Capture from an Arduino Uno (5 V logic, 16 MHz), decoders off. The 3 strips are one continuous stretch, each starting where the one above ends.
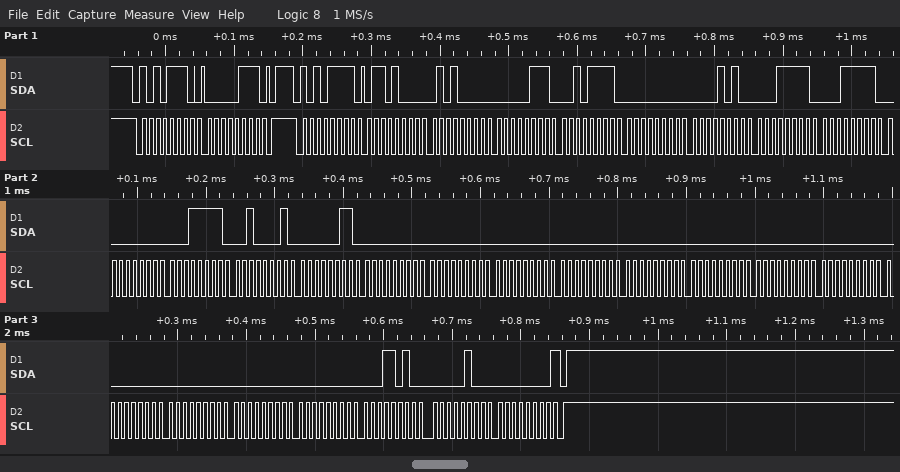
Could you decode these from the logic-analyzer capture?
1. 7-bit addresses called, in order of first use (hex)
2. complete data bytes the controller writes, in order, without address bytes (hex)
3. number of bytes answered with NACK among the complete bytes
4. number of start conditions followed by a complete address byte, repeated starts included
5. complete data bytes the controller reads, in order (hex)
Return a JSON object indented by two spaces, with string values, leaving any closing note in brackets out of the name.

{
  "7-bit addresses called, in order of first use": "0x57",
  "complete data bytes the controller writes, in order, without address bytes": "07",
  "number of bytes answered with NACK among the complete bytes": "1",
  "number of start conditions followed by a complete address byte, repeated starts included": "2",
  "complete data bytes the controller reads, in order": "68 50 07 2F 00 0A 1F 1F 00 1F 21 03 00 00 00 00 00 00 00 00 00 00 00 00 1A 04 00"
}
